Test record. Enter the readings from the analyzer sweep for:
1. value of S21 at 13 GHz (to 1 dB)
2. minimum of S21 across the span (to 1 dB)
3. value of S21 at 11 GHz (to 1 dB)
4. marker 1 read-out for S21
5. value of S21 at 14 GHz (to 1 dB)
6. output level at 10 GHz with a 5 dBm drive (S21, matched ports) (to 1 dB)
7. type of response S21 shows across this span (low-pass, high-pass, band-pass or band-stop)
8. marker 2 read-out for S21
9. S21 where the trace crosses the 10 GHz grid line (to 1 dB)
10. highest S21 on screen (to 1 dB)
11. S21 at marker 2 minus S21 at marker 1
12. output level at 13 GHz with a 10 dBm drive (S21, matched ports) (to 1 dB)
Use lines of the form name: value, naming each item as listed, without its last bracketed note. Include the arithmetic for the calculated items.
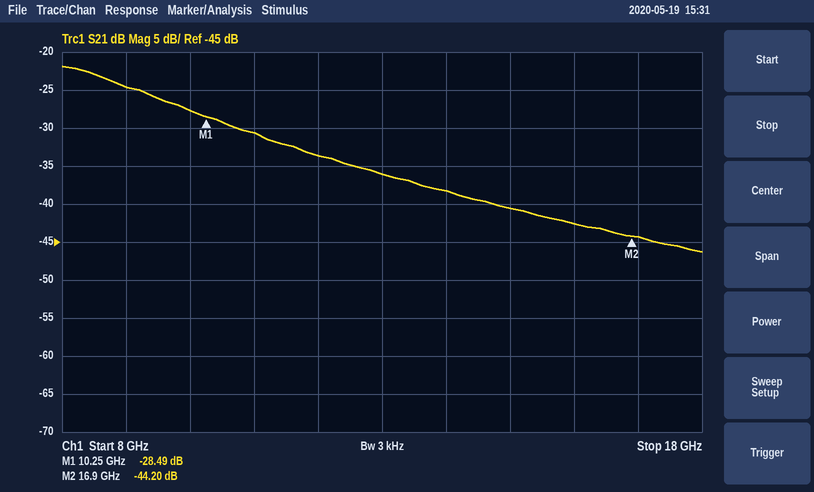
value of S21 at 13 GHz: -36 dB
minimum of S21 across the span: -46 dB
value of S21 at 11 GHz: -31 dB
marker 1 read-out for S21: -28.49 dB
value of S21 at 14 GHz: -38 dB
output level at 10 GHz with a 5 dBm drive (S21, matched ports): 5 dBm + (-28 dB) = -23 dBm
type of response S21 shows across this span: low-pass
marker 2 read-out for S21: -44.20 dB
S21 where the trace crosses the 10 GHz grid line: -28 dB
highest S21 on screen: -22 dB
S21 at marker 2 minus S21 at marker 1: -44.2 − (-28.49) = -15.71 dB
output level at 13 GHz with a 10 dBm drive (S21, matched ports): 10 dBm + (-36 dB) = -26 dBm
